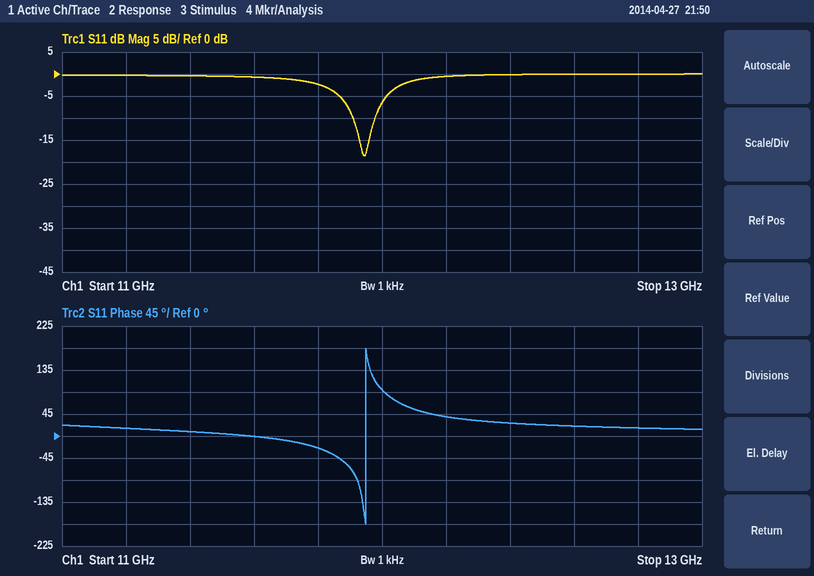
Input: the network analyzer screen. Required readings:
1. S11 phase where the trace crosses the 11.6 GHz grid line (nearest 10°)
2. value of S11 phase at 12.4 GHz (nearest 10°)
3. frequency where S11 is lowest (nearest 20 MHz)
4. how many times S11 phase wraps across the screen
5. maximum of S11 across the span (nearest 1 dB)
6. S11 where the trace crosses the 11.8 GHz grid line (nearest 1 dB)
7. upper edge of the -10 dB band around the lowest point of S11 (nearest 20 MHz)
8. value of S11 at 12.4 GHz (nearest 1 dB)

0°
30°
11.94 GHz
1
0 dB
-2 dB
11.98 GHz
0 dB
